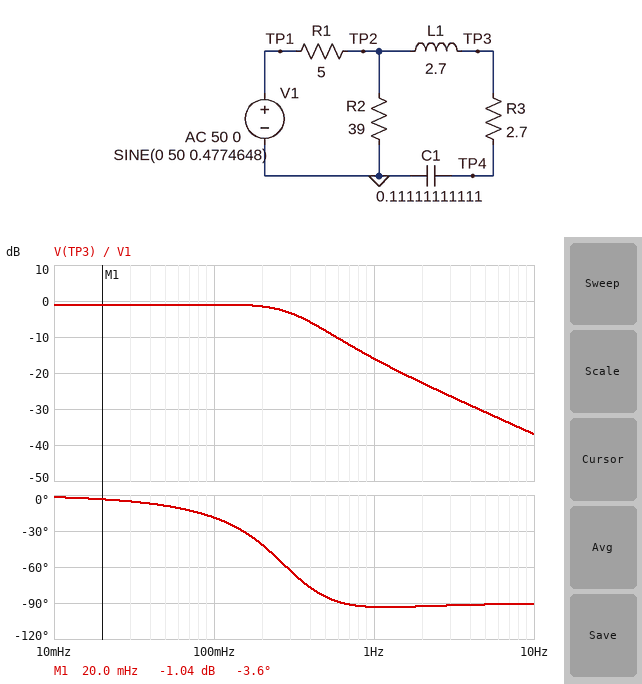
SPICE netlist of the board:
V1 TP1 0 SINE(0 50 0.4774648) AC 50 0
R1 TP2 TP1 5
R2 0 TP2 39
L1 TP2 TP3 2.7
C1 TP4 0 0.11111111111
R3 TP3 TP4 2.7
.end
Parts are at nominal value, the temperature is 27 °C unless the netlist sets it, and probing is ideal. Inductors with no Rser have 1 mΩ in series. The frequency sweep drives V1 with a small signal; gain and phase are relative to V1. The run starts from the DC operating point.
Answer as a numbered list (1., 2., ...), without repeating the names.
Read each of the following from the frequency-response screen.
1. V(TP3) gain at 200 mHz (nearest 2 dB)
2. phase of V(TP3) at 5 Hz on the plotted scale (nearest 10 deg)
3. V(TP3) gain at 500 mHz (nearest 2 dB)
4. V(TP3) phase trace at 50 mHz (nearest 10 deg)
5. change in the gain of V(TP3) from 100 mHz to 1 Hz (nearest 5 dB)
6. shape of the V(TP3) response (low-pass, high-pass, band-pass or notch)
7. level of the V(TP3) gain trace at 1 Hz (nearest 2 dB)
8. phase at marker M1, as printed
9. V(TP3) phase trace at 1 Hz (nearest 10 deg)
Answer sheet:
1. -2 dB
2. -90 deg
3. -8 dB
4. -10 deg
5. -15 dB
6. low-pass
7. -16 dB
8. -3.6 deg
9. -90 deg
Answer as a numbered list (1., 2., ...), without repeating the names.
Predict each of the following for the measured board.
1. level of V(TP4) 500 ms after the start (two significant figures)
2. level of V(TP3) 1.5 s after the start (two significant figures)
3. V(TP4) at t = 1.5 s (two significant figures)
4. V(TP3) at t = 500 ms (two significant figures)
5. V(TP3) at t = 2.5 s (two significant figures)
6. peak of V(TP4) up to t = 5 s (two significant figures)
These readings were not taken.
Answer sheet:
1. 5.8 V
2. 3.2 V
3. 15 V
4. 14 V
5. -5.6 V
6. 22 V
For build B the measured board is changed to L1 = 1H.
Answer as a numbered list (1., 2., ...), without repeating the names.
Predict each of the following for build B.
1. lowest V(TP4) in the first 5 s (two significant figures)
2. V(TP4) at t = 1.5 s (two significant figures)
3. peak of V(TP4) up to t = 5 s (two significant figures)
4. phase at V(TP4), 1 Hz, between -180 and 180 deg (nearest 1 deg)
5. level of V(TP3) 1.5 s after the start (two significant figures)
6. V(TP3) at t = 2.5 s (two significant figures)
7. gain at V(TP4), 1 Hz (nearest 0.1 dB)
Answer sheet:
1. -19 V
2. 6.2 V
3. 24 V
4. -124 deg
5. -11 V
6. 9.5 V
7. -16.6 dB
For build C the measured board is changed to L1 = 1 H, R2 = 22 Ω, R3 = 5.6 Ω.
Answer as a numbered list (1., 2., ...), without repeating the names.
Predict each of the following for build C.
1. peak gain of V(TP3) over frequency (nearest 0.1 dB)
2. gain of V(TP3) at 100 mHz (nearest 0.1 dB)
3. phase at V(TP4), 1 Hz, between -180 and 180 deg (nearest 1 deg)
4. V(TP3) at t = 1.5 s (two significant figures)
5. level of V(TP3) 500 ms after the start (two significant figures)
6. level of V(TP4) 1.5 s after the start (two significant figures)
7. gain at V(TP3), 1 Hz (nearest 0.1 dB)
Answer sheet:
1. -1.8 dB
2. -2.5 dB
3. -117 deg
4. -19 V
5. 26 V
6. 5.7 V
7. -7.2 dB
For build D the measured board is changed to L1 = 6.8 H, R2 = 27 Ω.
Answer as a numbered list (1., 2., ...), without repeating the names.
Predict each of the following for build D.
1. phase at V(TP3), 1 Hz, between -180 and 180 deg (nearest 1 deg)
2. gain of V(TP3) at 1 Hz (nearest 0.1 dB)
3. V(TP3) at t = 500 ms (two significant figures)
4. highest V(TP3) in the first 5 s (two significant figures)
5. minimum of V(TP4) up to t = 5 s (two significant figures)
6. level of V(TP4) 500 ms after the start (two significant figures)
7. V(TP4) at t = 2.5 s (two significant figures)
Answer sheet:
1. -108 deg
2. -24.2 dB
3. 6.9 V
4. 19 V
5. -8.7 V
6. 2.7 V
7. -4.4 V
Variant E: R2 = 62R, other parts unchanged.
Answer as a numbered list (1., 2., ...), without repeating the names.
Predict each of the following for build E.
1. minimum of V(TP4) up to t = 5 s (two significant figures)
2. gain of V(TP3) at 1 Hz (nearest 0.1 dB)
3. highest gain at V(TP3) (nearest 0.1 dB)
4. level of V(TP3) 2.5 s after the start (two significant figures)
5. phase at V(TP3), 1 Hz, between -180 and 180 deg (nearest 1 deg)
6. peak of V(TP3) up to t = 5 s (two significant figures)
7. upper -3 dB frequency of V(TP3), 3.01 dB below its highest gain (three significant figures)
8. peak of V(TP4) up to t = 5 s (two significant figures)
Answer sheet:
1. -16 V
2. -15.7 dB
3. -0.7 dB
4. -5.4 V
5. -93 deg
6. 27 V
7. 320 mHz
8. 23 V
